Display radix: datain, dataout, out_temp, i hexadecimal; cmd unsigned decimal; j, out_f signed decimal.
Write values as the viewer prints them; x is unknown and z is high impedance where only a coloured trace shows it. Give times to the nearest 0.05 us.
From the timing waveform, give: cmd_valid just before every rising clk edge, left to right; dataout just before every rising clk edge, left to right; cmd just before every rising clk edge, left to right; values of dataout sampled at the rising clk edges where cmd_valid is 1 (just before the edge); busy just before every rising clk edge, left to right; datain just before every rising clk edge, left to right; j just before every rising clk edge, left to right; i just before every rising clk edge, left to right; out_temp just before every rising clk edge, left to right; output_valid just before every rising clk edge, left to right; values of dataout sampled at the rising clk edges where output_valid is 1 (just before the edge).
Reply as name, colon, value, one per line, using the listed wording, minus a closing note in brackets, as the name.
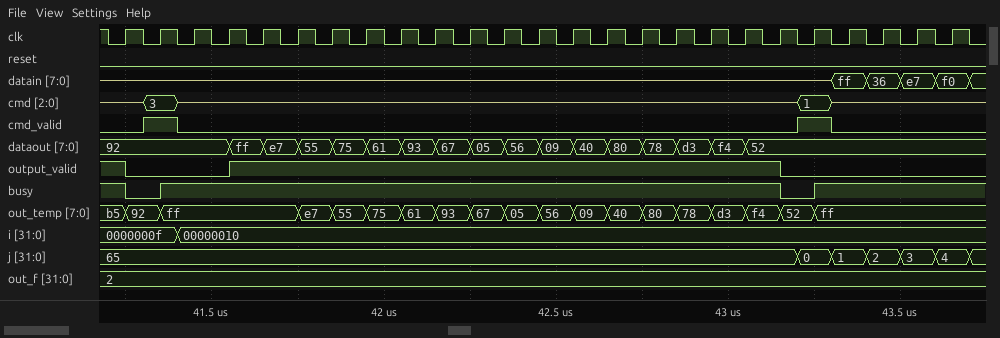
cmd_valid just before every rising clk edge, left to right: 0 1 0 0 0 0 0 0 0 0 0 0 0 0 0 0 0 0 0 0 1 0 0 0 0
dataout just before every rising clk edge, left to right: 92, 92, 92, 92, ff, e7, 55, 75, 61, 93, 67, 05, 56, 09, 40, 80, 78, d3, f4, 52, 52, 52, 52, 52, 52
cmd just before every rising clk edge, left to right: z, 3, z, z, z, z, z, z, z, z, z, z, z, z, z, z, z, z, z, z, 1, z, z, z, z
values of dataout sampled at the rising clk edges where cmd_valid is 1: 92, 52
busy just before every rising clk edge, left to right: 1 0 1 1 1 1 1 1 1 1 1 1 1 1 1 1 1 1 1 1 0 1 1 1 1
datain just before every rising clk edge, left to right: z, z, z, z, z, z, z, z, z, z, z, z, z, z, z, z, z, z, z, z, z, ff, 36, e7, f0
j just before every rising clk edge, left to right: 65, 65, 65, 65, 65, 65, 65, 65, 65, 65, 65, 65, 65, 65, 65, 65, 65, 65, 65, 65, 0, 1, 2, 3, 4
i just before every rising clk edge, left to right: 0000000f, 0000000f, 00000010, 00000010, 00000010, 00000010, 00000010, 00000010, 00000010, 00000010, 00000010, 00000010, 00000010, 00000010, 00000010, 00000010, 00000010, 00000010, 00000010, 00000010, 00000010, 00000010, 00000010, 00000010, 00000010
out_temp just before every rising clk edge, left to right: b5, 92, ff, ff, ff, ff, e7, 55, 75, 61, 93, 67, 05, 56, 09, 40, 80, 78, d3, f4, 52, ff, ff, ff, ff
output_valid just before every rising clk edge, left to right: 1 0 0 0 1 1 1 1 1 1 1 1 1 1 1 1 1 1 1 1 0 0 0 0 0
values of dataout sampled at the rising clk edges where output_valid is 1: 92, ff, e7, 55, 75, 61, 93, 67, 05, 56, 09, 40, 80, 78, d3, f4, 52
